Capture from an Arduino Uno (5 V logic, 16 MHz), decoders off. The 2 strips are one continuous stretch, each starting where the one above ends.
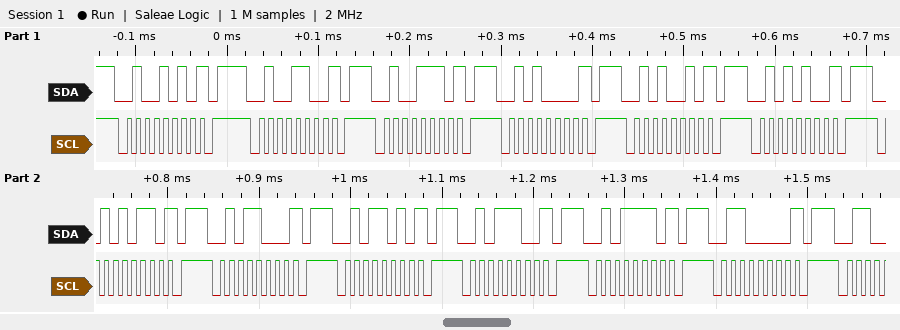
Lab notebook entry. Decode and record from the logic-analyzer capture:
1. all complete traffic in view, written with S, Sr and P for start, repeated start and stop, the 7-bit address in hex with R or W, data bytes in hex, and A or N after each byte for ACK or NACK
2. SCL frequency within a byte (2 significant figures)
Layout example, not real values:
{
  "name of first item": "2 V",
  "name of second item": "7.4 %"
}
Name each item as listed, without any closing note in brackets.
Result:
{
  "all complete traffic in view, written with S, Sr and P for start, repeated start and stop, the 7-bit address in hex with R or W, data bytes in hex, and A or N after each byte for ACK or NACK": "S 25W N P S 26W N P S 27W N P S 28W N P S 29W N P S 2AW N P S 2BW N P S 2CW N P S 2DW N P S 2EW N P S 2FW N P S 30W N P",
  "SCL frequency within a byte": "100 kHz"
}
